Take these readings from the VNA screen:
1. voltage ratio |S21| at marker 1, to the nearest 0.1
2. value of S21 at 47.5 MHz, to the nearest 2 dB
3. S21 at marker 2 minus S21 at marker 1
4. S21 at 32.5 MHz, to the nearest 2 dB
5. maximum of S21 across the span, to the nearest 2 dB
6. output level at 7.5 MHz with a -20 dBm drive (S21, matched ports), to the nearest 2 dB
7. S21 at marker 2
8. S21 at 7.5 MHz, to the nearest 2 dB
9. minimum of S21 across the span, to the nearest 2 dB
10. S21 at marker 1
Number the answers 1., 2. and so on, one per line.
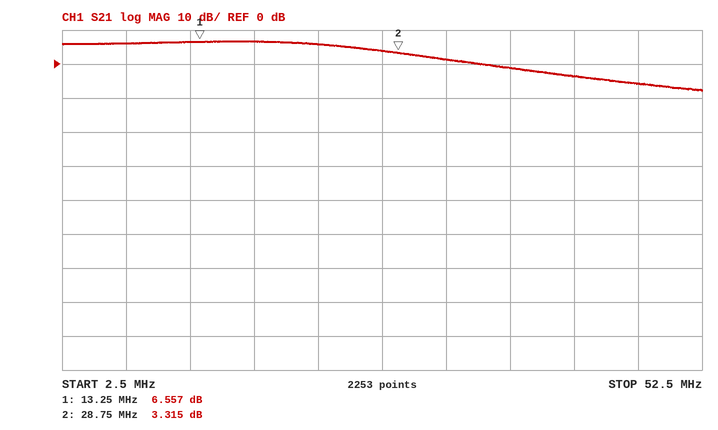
1. 2.1
2. -6 dB
3. -3.242 dB
4. 2 dB
5. 6 dB
6. -14 dBm
7. 3.315 dB
8. 6 dB
9. -8 dB
10. 6.557 dB
